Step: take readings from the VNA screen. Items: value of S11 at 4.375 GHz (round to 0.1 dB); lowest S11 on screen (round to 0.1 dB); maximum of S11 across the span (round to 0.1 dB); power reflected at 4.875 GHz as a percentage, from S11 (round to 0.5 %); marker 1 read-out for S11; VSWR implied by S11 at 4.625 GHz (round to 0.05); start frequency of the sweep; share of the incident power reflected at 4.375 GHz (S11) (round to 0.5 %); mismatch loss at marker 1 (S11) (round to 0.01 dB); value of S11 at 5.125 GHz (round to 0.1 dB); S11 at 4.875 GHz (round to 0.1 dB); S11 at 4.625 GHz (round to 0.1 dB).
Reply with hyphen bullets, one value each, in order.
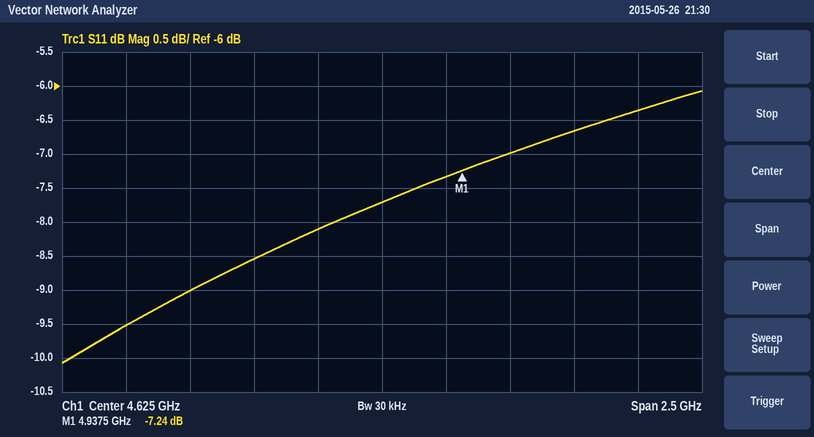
- -8.1 dB
- -10.1 dB
- -6.1 dB
- 18.5 %
- -7.24 dB
- 2.40
- 3.375 GHz
- 15.5 %
- 0.91 dB
- -7.0 dB
- -7.3 dB
- -7.7 dB
